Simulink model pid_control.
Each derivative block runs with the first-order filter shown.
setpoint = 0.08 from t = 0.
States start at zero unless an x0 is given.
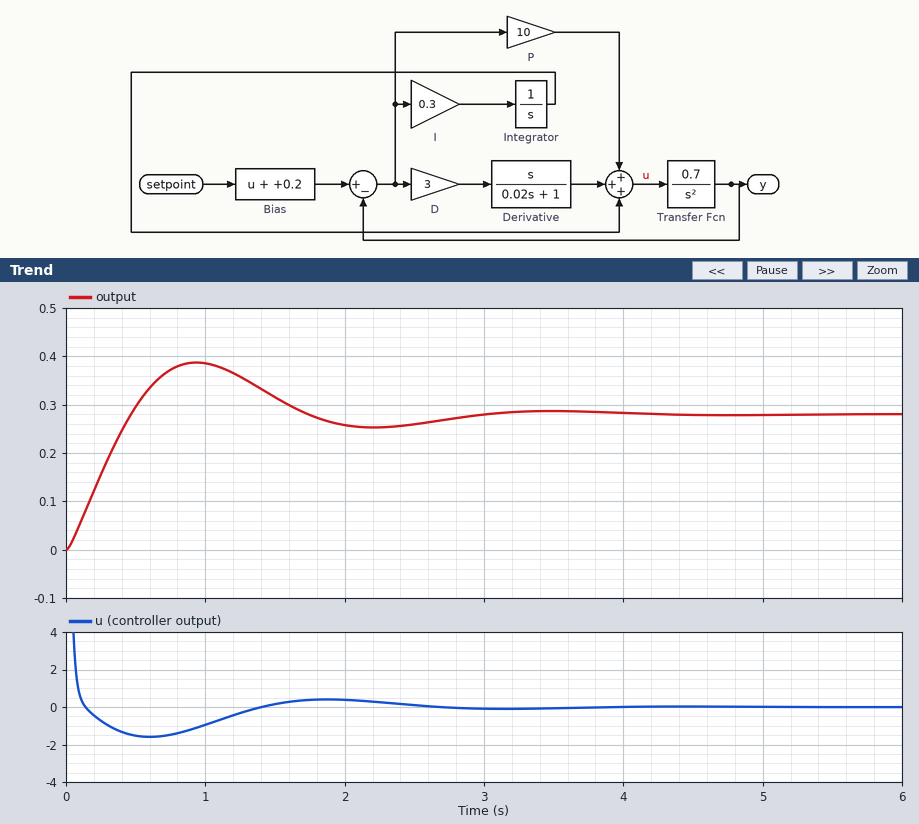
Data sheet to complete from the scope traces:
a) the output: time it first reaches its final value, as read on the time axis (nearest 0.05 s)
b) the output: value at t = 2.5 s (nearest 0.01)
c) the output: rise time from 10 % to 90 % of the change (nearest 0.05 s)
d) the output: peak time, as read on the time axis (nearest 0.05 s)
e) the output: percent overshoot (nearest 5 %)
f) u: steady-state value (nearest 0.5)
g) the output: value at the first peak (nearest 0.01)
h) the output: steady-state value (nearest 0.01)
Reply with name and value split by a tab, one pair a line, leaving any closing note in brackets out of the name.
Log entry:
the output: time it first reaches its final value, as read on the time axis	0.45 s
the output: value at t = 2.5 s	0.26
the output: rise time from 10 % to 90 % of the change	0.35 s
the output: peak time, as read on the time axis	0.95 s
the output: percent overshoot	40 %
u: steady-state value	0.0
the output: value at the first peak	0.39
the output: steady-state value	0.28
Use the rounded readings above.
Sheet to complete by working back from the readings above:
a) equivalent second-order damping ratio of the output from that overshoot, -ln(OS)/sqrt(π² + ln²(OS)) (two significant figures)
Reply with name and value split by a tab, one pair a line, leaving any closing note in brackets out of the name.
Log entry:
equivalent second-order damping ratio of the output from that overshoot, -ln(OS)/sqrt(π² + ln²(OS))	0.28
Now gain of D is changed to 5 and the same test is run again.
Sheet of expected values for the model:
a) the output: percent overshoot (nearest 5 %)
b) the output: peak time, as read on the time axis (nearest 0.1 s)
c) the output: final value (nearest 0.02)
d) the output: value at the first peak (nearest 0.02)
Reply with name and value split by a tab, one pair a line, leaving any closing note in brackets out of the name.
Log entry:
the output: percent overshoot	25 %
the output: peak time, as read on the time axis	0.8 s
the output: final value	0.28
the output: value at the first peak	0.34
